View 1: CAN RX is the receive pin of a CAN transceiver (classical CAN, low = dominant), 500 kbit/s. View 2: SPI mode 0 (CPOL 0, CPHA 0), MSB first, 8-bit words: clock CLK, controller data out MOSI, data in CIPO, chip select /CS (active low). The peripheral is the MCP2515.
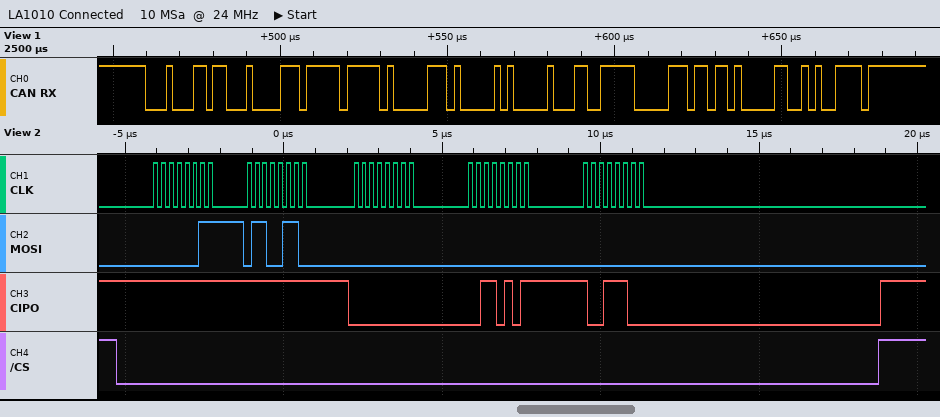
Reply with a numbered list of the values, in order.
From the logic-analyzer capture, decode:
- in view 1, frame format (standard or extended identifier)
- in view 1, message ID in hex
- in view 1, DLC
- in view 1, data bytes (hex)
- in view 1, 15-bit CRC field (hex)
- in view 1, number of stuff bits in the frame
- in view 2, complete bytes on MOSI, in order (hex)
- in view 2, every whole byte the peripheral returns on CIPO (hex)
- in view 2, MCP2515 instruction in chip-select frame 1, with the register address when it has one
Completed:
1. standard
2. 0x11B
3. 8
4. 77 FF 06 81 00 CF 86 DA
5. 0x04A7
6. 8
7. 03 66 00 00 00
8. FF FF 00 35 9C
9. READ 0x66
